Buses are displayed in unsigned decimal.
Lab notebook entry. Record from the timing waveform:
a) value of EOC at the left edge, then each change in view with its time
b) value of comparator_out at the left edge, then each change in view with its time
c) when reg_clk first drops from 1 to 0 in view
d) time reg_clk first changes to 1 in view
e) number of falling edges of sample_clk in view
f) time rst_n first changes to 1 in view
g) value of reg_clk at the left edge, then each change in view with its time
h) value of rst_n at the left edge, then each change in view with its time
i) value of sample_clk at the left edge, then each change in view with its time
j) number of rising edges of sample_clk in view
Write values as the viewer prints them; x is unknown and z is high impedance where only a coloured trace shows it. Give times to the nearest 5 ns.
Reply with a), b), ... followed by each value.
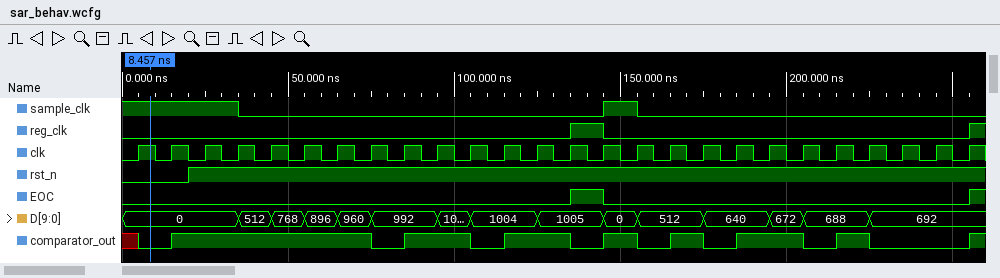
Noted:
a) 0, 1 at 135 ns, 0 at 145 ns, 1 at 255 ns
b) x, 0 at 5 ns, 1 at 15 ns, 0 at 75 ns, 1 at 85 ns, 0 at 105 ns, 1 at 115 ns, 0 at 135 ns, 1 at 145 ns, 0 at 155 ns, 1 at 165 ns, 0 at 175 ns, 1 at 185 ns, 0 at 205 ns, 1 at 215 ns, 0 at 225 ns, 1 at 255 ns
c) 145 ns
d) 135 ns
e) 2
f) 20 ns
g) 0, 1 at 135 ns, 0 at 145 ns, 1 at 255 ns
h) 0, 1 at 20 ns
i) 1, 0 at 35 ns, 1 at 145 ns, 0 at 155 ns
j) 1
